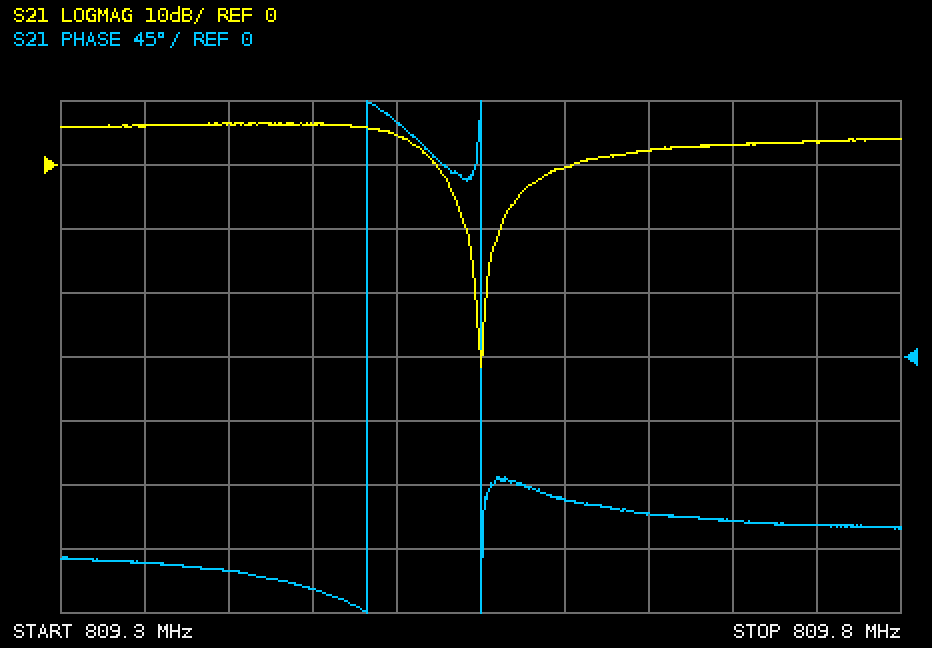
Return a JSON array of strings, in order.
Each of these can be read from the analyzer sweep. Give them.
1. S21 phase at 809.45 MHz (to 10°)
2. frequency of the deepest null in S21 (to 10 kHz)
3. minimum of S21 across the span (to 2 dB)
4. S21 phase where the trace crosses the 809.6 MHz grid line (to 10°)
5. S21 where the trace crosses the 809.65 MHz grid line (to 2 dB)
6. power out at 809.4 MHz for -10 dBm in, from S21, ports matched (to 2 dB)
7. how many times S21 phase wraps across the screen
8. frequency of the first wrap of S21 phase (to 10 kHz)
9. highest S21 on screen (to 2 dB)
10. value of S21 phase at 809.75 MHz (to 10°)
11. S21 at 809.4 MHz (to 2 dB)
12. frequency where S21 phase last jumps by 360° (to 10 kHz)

["-160°", "809.55 MHz", "-32 dB", "-100°", "2 dB", "-4 dBm", "2", "809.48 MHz", "6 dB", "-120°", "6 dB", "809.55 MHz"]
